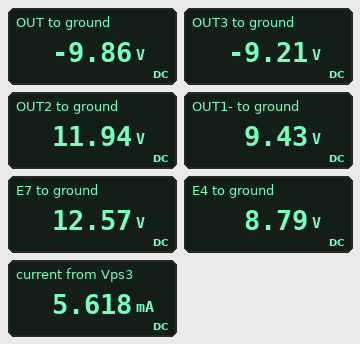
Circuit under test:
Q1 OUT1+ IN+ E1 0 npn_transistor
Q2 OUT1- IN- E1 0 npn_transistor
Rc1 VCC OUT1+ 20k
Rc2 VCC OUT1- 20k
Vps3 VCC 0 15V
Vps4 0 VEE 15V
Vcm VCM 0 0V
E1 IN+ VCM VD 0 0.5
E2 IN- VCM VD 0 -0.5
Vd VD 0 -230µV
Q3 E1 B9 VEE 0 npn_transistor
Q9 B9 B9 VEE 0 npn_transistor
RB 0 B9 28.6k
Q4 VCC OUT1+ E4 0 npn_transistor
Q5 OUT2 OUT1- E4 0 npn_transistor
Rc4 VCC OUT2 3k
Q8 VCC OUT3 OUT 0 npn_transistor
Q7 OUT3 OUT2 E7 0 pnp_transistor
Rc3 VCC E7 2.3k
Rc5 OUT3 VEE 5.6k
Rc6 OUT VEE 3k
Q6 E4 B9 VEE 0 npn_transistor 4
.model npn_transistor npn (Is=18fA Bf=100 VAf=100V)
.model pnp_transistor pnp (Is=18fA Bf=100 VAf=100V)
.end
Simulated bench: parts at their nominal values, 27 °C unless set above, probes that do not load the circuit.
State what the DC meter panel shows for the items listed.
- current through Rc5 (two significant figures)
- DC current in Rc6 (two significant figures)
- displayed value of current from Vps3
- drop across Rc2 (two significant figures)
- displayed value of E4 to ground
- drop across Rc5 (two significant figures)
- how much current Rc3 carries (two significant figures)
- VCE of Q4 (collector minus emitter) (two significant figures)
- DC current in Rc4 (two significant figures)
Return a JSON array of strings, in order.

["1.0 mA", "1.7 mA", "5.618 mA", "5.6 V", "8.79 V", "5.8 V", "1.1 mA", "6.2 V", "1.0 mA"]
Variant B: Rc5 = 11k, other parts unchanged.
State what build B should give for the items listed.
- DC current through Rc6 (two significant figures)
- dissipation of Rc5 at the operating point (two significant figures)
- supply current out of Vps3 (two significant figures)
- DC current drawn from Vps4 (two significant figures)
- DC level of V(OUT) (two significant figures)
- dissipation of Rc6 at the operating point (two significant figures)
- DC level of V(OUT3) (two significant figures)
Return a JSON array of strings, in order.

["3.5 mA", "11 mW", "7.4 mA", "7.9 mA", "-4.5 V", "37 mW", "-3.8 V"]
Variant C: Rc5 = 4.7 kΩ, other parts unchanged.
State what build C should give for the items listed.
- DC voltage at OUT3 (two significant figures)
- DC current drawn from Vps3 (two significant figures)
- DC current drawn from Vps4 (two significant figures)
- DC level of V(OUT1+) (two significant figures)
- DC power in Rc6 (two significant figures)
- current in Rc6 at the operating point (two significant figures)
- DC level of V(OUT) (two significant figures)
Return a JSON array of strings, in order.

["-10 V", "5.3 mA", "5.8 mA", "9.4 V", "6.0 mW", "1.4 mA", "-11 V"]
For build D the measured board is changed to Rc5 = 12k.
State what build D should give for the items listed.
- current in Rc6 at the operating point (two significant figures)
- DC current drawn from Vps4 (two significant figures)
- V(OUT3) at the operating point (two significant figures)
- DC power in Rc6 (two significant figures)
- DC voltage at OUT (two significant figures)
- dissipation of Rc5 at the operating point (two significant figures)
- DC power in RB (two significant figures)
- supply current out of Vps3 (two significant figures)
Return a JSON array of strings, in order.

["3.8 mA", "8.2 mA", "-2.8 V", "44 mW", "-3.5 V", "12 mW", "7.2 mW", "7.7 mA"]
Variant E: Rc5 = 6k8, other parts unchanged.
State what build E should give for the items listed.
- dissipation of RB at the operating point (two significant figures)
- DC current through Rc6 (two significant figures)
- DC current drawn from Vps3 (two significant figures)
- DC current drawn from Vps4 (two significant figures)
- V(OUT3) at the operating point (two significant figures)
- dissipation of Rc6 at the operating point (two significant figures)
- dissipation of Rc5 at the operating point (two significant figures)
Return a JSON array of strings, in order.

["7.2 mW", "2.1 mA", "6.0 mA", "6.5 mA", "-8.0 V", "13 mW", "7.2 mW"]
